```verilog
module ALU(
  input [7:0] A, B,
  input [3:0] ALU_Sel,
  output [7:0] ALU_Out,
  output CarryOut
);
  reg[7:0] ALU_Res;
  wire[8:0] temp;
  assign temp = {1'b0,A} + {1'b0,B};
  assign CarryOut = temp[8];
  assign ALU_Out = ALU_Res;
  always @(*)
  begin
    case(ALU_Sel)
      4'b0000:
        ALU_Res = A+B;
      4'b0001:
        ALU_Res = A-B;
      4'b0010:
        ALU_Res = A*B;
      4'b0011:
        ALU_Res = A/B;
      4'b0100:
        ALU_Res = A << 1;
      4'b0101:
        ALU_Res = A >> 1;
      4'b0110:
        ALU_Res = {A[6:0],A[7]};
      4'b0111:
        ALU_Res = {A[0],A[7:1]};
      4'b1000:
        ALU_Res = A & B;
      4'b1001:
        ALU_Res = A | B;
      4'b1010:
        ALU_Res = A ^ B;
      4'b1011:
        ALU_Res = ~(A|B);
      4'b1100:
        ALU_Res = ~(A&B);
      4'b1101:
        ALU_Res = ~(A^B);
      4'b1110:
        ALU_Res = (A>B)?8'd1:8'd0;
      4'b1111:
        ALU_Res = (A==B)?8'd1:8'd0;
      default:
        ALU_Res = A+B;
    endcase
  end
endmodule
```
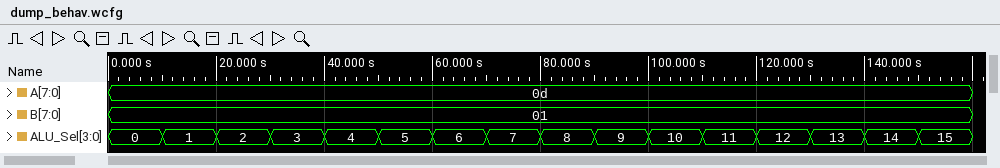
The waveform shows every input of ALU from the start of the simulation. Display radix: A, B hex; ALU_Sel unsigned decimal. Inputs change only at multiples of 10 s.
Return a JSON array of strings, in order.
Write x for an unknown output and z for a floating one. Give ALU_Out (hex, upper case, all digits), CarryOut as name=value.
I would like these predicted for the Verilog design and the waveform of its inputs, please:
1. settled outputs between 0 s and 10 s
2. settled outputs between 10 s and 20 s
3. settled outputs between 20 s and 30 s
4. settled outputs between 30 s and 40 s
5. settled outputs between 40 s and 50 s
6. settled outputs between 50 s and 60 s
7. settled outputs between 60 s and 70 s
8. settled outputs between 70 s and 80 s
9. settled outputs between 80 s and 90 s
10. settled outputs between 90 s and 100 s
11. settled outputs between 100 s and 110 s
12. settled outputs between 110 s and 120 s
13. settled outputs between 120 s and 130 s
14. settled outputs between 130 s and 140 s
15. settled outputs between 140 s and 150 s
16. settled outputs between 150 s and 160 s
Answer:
["ALU_Out=0E, CarryOut=0", "ALU_Out=0C, CarryOut=0", "ALU_Out=0D, CarryOut=0", "ALU_Out=0D, CarryOut=0", "ALU_Out=1A, CarryOut=0", "ALU_Out=06, CarryOut=0", "ALU_Out=1A, CarryOut=0", "ALU_Out=86, CarryOut=0", "ALU_Out=01, CarryOut=0", "ALU_Out=0D, CarryOut=0", "ALU_Out=0C, CarryOut=0", "ALU_Out=F2, CarryOut=0", "ALU_Out=FE, CarryOut=0", "ALU_Out=F3, CarryOut=0", "ALU_Out=01, CarryOut=0", "ALU_Out=00, CarryOut=0"]
